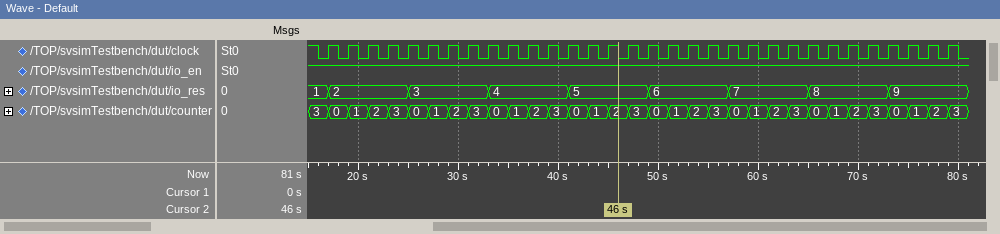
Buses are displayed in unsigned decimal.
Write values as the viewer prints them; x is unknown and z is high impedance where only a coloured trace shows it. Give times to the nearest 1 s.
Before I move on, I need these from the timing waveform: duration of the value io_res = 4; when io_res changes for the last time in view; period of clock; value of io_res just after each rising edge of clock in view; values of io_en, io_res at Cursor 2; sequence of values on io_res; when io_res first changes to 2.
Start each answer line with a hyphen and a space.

- 8 s
- 73 s
- 2 s
- 2, 2, 2, 2, 3, 3, 3, 3, 4, 4, 4, 4, 5, 5, 5, 5, 6, 6, 6, 6, 7, 7, 7, 7, 8, 8, 8, 8, 9, 9, 9, 9
- io_en=1, io_res=5
- 1, 2, 3, 4, 5, 6, 7, 8, 9
- 17 s
